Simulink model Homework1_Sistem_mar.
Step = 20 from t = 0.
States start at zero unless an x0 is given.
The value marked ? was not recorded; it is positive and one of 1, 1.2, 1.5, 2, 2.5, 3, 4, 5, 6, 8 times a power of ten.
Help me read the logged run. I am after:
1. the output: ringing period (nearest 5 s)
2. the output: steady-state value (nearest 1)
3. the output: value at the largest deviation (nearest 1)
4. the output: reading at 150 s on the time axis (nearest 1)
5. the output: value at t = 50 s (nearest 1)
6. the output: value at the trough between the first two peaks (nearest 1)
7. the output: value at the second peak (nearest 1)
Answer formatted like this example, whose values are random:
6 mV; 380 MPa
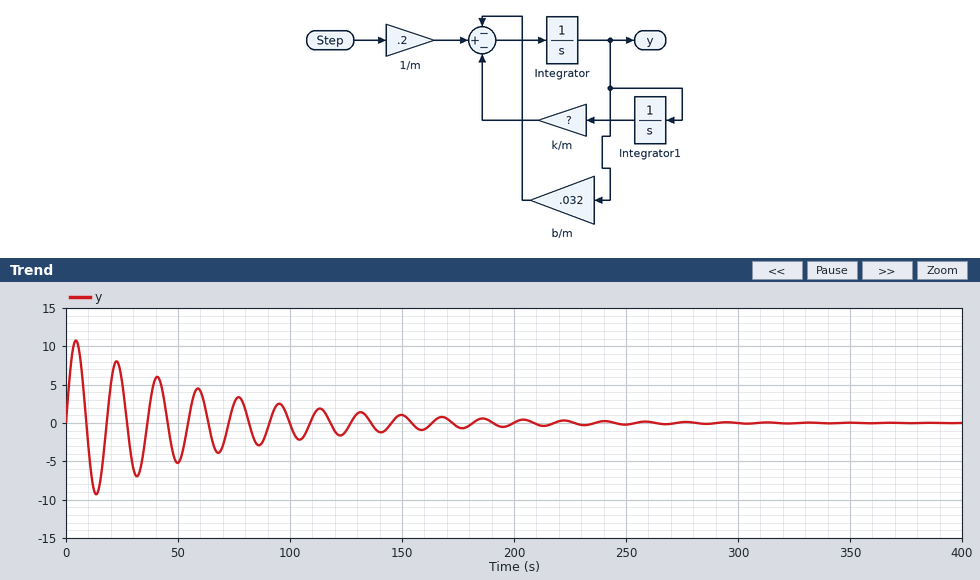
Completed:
20 s; 0; 11; 1; -5; -9; 8
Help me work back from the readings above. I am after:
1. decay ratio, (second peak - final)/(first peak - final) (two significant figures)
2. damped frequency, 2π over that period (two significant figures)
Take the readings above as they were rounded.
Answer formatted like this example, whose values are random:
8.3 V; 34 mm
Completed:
0.73; 0.31 rad/s
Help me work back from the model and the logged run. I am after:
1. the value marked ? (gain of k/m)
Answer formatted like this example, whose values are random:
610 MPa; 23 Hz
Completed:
0.12
